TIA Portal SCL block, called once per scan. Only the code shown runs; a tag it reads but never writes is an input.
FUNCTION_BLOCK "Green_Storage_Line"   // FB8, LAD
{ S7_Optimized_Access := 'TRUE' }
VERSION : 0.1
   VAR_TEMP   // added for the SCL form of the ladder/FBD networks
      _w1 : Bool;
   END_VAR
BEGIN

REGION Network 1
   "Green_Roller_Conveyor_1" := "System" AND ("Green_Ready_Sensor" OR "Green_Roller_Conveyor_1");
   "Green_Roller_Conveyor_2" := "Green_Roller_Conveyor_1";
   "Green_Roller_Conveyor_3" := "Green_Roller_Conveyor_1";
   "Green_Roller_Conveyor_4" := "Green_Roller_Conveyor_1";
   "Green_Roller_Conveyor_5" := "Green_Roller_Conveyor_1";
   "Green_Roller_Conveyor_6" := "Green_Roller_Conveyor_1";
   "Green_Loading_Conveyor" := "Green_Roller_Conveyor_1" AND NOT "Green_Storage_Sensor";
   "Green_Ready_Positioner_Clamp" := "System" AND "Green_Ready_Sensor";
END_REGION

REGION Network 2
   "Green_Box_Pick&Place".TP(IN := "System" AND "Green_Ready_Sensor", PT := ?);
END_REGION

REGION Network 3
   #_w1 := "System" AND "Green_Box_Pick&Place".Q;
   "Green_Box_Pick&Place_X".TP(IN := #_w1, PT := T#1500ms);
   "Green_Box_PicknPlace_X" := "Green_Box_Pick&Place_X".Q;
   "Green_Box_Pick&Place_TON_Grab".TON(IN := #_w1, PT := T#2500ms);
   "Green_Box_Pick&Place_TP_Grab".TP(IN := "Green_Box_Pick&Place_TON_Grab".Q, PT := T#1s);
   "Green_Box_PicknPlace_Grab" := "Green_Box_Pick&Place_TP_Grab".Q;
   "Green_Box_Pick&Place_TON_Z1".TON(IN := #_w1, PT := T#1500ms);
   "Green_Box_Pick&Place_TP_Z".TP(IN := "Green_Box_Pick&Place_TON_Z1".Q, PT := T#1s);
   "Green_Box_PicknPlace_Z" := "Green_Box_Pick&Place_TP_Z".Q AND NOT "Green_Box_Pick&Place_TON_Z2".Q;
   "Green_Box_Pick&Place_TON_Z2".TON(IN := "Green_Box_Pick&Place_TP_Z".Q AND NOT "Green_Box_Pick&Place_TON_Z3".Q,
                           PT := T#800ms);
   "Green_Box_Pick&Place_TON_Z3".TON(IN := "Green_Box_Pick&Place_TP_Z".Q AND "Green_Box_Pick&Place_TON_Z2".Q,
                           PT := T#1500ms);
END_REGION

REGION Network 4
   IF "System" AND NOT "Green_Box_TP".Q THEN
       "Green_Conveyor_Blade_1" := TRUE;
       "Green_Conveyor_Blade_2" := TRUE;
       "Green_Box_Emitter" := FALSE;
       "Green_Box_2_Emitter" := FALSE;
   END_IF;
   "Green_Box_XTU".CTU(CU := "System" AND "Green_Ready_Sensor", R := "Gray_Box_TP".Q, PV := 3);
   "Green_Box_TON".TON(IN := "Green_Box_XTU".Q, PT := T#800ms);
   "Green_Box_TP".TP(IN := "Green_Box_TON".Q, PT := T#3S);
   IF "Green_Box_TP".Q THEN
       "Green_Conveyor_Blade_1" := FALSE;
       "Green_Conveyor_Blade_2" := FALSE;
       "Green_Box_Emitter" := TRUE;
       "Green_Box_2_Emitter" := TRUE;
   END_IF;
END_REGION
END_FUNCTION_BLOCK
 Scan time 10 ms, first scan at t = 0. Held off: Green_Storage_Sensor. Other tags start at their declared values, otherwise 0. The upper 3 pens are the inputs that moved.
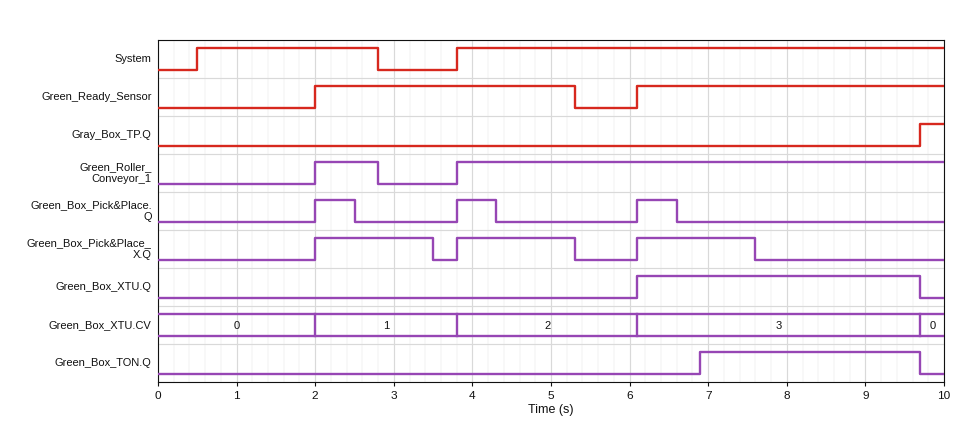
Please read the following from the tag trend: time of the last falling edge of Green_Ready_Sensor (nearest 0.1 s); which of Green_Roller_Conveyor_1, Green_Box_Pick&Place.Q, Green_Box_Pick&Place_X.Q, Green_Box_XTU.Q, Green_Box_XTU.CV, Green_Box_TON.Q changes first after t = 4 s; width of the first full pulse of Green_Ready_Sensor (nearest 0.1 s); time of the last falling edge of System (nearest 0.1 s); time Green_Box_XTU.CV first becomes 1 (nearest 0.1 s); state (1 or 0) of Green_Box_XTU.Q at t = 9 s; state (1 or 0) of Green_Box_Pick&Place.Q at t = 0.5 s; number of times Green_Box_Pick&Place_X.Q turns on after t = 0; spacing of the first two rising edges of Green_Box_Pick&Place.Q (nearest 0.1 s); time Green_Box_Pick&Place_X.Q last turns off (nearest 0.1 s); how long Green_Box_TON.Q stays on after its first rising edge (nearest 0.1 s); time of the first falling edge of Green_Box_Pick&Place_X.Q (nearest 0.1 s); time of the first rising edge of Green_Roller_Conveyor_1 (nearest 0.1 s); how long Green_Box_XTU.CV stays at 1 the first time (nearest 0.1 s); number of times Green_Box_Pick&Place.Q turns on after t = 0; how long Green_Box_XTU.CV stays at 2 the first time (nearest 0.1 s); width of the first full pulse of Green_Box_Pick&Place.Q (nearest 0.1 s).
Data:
5.3 s
Green_Box_Pick&Place.Q
3.3 s
2.8 s
2.0 s
1
0
3
1.8 s
7.6 s
2.8 s
3.5 s
2.0 s
1.8 s
3
2.3 s
0.5 s
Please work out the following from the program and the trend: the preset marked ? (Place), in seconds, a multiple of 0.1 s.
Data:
0.5 s
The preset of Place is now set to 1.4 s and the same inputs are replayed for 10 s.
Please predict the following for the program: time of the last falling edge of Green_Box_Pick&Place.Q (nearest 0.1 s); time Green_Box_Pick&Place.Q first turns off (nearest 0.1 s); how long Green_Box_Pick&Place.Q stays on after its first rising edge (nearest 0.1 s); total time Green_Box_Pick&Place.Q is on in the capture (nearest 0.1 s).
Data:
7.5 s
3.4 s
1.4 s
4.2 s
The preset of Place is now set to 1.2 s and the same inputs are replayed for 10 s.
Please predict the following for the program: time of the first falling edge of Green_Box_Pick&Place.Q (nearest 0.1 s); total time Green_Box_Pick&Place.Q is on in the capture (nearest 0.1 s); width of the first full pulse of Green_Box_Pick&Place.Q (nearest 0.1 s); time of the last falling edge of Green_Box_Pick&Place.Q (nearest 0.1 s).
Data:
3.2 s
3.6 s
1.2 s
7.3 s
